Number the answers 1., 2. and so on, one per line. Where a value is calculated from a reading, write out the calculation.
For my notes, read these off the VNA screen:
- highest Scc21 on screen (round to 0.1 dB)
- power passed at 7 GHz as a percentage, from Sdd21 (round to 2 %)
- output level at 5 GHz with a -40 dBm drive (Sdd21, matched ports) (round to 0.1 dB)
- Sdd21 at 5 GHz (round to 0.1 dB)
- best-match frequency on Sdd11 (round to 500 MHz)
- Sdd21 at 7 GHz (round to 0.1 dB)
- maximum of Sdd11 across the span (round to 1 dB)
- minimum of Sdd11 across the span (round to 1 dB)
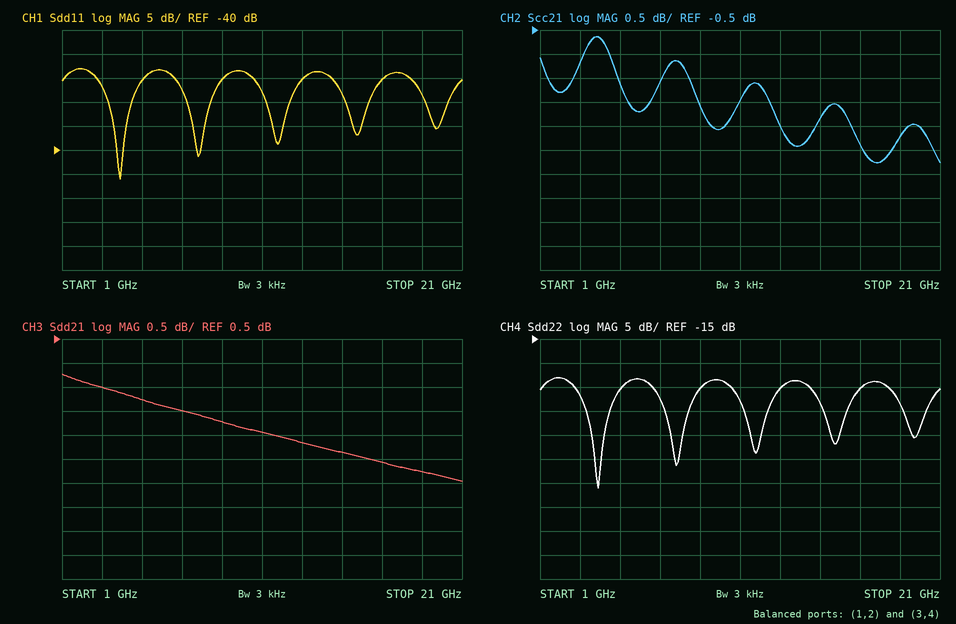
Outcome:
1. -0.6 dB
2. 10^(-1/10) ≈ 79.4 %, so 80 % to the nearest 2 %
3. -40 dBm + (-0.8 dB) = -40.8 dBm
4. -0.8 dB
5. 4.0 GHz
6. -1.0 dB
7. -23 dB
8. -46 dB
